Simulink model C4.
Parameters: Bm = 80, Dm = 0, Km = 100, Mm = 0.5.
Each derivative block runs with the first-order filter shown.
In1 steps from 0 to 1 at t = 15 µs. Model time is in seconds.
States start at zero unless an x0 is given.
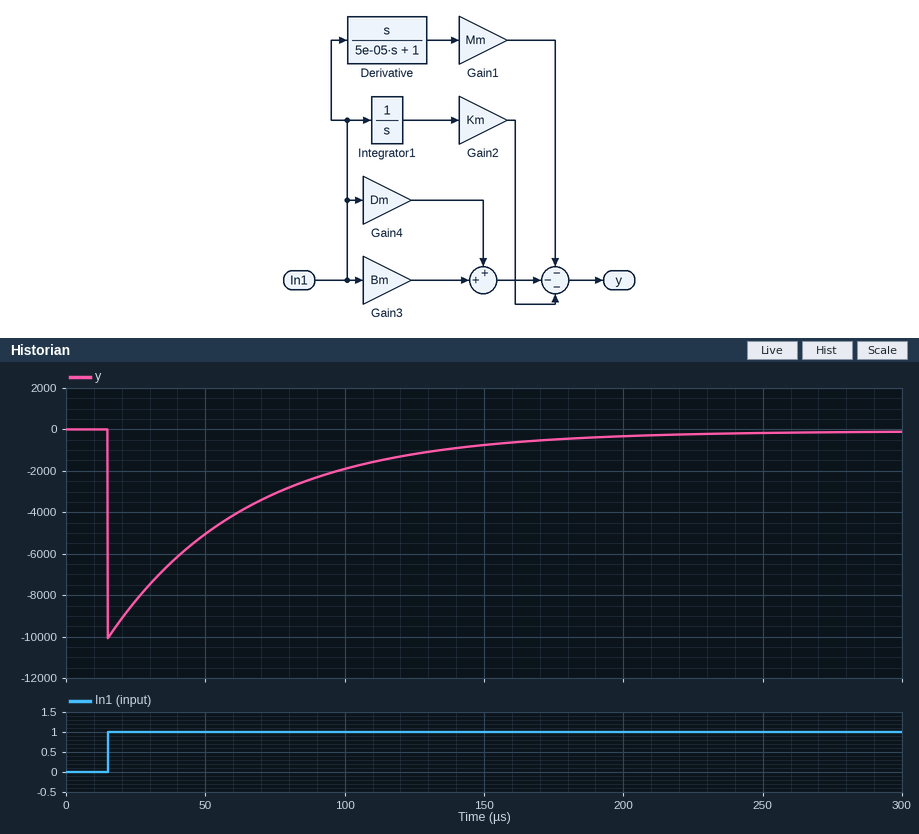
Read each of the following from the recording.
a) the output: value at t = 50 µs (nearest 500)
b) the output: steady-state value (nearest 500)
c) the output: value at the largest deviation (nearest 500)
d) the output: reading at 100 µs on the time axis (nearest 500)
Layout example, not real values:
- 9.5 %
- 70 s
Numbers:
- -5000
- 0
- -10000
- -2000
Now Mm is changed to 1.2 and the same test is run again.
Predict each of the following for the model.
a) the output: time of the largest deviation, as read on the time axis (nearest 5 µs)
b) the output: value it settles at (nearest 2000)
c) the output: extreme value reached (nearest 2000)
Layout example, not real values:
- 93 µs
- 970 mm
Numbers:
- 15 µs
- 0
- -24000
